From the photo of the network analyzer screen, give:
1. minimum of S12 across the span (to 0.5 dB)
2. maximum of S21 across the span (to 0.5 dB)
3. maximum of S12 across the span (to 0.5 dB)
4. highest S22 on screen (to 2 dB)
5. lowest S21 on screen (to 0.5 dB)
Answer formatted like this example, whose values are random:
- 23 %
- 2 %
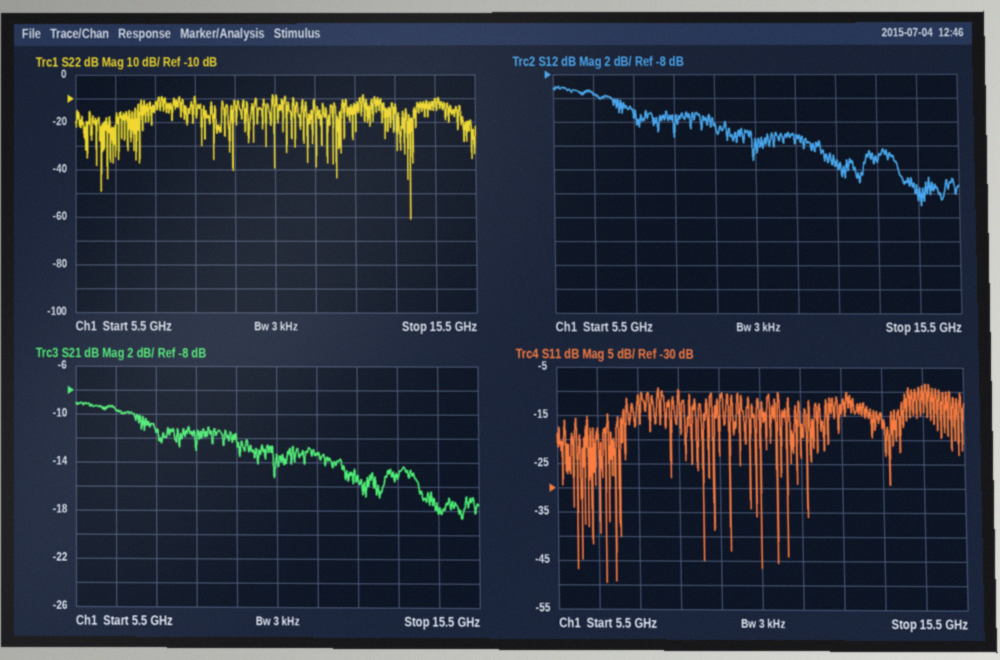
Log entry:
- -19.0 dB
- -9.0 dB
- -9.0 dB
- -8 dB
- -18.5 dB
